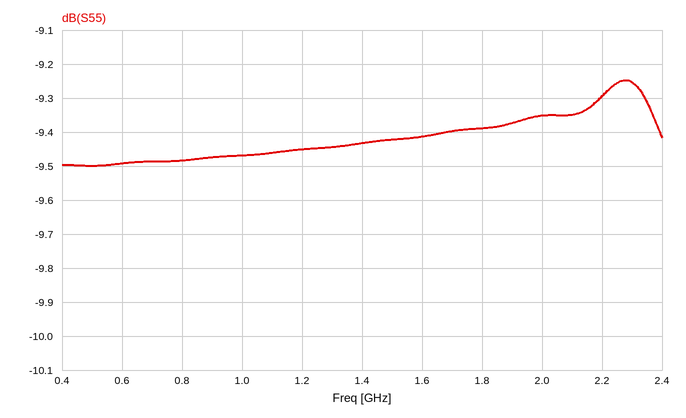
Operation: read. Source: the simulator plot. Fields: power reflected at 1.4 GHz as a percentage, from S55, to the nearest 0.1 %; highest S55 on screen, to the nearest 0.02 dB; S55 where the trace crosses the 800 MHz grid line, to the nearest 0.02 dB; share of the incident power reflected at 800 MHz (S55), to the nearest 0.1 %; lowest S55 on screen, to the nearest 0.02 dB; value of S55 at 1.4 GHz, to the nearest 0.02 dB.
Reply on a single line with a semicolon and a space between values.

11.4 %; -9.24 dB; -9.48 dB; 11.3 %; -9.50 dB; -9.44 dB
